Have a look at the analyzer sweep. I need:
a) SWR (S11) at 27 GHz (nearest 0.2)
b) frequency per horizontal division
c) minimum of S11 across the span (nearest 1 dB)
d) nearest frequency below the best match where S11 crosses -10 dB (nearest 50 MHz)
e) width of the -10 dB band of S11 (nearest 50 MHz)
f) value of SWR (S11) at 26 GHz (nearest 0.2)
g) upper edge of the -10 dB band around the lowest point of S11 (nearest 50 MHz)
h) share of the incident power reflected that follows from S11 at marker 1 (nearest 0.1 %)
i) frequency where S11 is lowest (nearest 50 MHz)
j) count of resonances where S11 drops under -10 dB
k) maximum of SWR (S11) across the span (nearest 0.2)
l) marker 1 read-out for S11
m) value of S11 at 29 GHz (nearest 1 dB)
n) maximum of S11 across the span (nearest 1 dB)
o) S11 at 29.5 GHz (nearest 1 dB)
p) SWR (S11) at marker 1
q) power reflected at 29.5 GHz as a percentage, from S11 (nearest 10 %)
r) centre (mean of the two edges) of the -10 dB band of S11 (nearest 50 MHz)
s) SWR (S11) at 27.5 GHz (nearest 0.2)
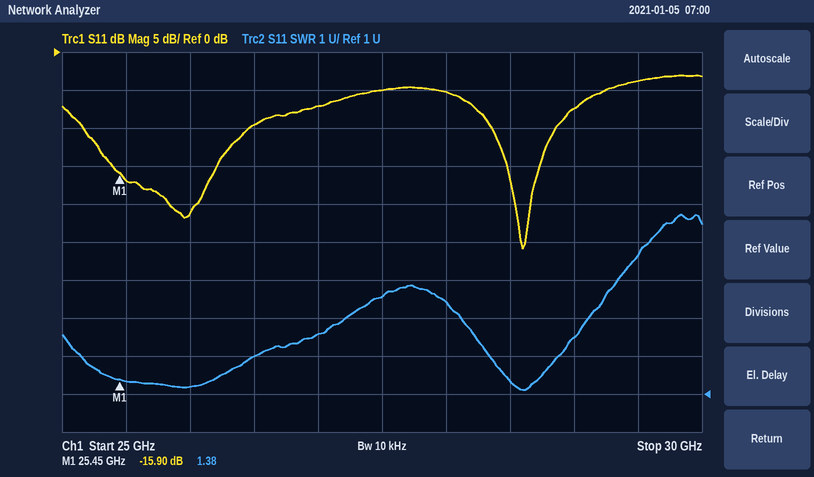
2.6
500 MHz
-26 dB
28.35 GHz
500 MHz
1.2
28.85 GHz
2.6 %
28.60 GHz
2
5.8
-15.90 dB
-7 dB
-3 dB
-4 dB
1.38
40 %
28.60 GHz
3.6
